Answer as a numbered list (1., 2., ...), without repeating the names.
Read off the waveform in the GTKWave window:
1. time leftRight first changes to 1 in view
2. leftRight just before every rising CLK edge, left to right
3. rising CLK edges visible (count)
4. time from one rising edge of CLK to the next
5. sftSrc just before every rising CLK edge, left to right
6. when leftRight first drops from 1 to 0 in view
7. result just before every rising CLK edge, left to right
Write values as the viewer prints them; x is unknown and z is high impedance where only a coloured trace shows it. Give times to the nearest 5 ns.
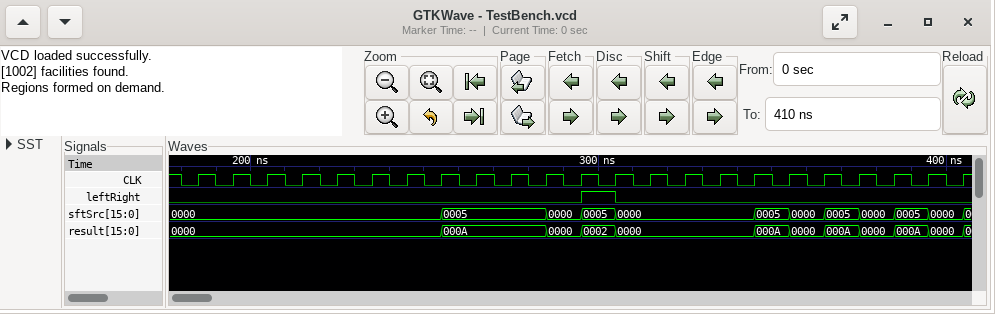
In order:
1. 295 ns
2. 0 0 0 0 0 0 0 0 0 0 0 0 1 0 0 0 0 0 0 0 0 0 0
3. 23
4. 10 ns
5. 0000, 0000, 0000, 0000, 0000, 0000, 0000, 0000, 0005, 0005, 0005, 0000, 0005, 0000, 0000, 0000, 0000, 0005, 0000, 0005, 0000, 0005, 0000
6. 305 ns
7. 0000, 0000, 0000, 0000, 0000, 0000, 0000, 0000, 000A, 000A, 000A, 0000, 0002, 0000, 0000, 0000, 0000, 000A, 0000, 000A, 0000, 000A, 0000
